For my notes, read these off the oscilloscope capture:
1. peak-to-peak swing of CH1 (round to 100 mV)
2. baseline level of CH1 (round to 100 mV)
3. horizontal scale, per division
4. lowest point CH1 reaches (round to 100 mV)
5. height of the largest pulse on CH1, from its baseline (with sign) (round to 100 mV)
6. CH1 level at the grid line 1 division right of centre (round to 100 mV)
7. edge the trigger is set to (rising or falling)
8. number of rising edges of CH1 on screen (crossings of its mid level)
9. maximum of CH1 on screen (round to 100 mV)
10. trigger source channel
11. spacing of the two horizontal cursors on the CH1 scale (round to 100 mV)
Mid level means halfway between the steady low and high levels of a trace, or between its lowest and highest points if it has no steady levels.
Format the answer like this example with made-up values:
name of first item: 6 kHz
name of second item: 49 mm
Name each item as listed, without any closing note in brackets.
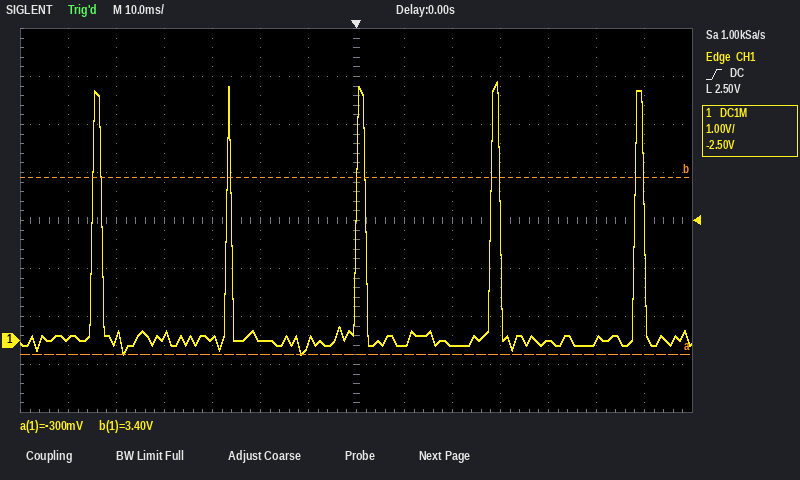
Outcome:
peak-to-peak swing of CH1: 5.7 V
baseline level of CH1: 0.0 V
horizontal scale, per division: 10 ms
lowest point CH1 reaches: -300 mV
height of the largest pulse on CH1, from its baseline (with sign): +5.4 V
CH1 level at the grid line 1 division right of centre: -100 mV
edge the trigger is set to: rising
number of rising edges of CH1 on screen: 5
maximum of CH1 on screen: 5.4 V
trigger source channel: CH1
spacing of the two horizontal cursors on the CH1 scale: 3.7 V
